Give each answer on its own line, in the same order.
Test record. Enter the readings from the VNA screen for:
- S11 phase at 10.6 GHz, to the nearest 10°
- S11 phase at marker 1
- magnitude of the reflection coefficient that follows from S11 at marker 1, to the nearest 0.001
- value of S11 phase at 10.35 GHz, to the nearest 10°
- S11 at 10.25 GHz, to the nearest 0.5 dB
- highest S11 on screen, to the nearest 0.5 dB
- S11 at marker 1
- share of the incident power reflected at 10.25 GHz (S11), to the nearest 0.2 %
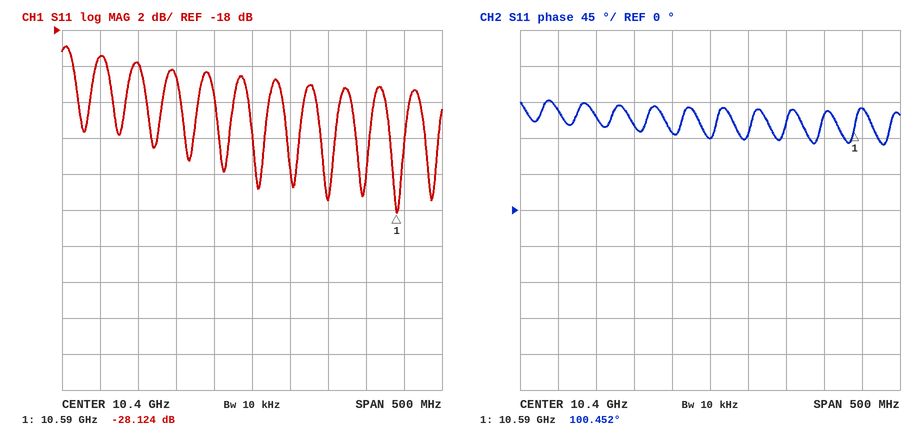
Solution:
130°
100.452°
0.039
100°
-20.0 dB
-19.0 dB
-28.124 dB
1.0 %
